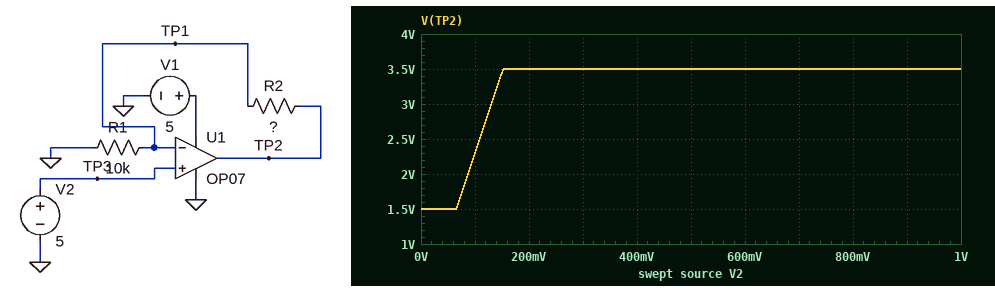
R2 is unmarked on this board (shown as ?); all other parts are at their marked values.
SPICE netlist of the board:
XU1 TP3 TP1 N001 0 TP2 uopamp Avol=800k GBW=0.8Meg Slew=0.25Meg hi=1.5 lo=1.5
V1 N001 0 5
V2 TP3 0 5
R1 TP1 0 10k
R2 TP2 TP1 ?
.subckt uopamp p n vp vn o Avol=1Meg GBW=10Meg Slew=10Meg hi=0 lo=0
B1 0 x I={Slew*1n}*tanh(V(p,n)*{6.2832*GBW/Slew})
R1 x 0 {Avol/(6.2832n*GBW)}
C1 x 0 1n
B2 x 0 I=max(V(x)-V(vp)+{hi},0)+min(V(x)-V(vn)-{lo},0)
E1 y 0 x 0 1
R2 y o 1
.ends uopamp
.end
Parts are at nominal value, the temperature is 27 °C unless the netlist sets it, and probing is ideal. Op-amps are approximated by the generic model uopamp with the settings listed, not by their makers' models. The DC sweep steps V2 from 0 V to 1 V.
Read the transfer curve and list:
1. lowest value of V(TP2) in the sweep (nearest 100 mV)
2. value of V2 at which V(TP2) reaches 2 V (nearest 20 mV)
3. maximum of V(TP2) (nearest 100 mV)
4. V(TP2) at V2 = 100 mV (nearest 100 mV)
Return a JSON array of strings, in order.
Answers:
["1.5 V", "80 mV", "3.5 V", "2.3 V"]
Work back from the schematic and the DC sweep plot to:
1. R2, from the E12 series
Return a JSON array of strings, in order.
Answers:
["220 kΩ"]
